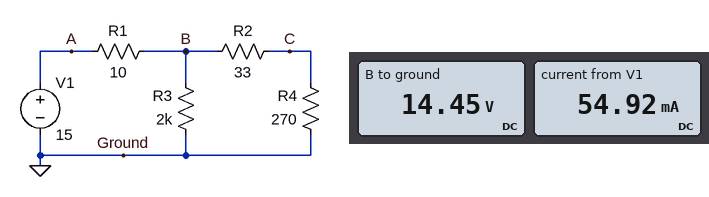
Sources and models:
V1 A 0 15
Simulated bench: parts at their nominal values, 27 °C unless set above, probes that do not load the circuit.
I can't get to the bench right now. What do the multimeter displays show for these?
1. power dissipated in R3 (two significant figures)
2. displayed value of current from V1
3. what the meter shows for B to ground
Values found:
100 mW
54.92 mA
14.45 V
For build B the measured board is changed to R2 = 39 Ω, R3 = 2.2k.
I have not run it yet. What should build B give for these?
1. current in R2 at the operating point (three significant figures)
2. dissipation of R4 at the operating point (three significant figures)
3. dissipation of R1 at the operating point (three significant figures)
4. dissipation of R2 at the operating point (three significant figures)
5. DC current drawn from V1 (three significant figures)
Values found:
46.8 mA
592 mW
28.5 mW
85.5 mW
53.4 mA
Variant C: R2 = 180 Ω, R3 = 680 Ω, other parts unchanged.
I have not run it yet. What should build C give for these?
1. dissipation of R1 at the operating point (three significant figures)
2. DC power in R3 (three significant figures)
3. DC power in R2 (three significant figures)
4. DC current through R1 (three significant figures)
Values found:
28.5 mW
308 mW
186 mW
53.4 mA
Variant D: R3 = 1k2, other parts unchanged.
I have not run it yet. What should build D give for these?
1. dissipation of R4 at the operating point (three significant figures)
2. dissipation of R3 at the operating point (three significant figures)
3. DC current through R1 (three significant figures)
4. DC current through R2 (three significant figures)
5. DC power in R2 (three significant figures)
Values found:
610 mW
173 mW
59.5 mA
47.5 mA
74.6 mW
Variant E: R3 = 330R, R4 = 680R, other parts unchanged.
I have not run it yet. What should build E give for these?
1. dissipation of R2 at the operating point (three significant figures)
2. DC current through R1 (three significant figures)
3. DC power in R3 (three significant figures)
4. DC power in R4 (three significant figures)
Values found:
13.4 mW
63.7 mA
625 mW
276 mW
